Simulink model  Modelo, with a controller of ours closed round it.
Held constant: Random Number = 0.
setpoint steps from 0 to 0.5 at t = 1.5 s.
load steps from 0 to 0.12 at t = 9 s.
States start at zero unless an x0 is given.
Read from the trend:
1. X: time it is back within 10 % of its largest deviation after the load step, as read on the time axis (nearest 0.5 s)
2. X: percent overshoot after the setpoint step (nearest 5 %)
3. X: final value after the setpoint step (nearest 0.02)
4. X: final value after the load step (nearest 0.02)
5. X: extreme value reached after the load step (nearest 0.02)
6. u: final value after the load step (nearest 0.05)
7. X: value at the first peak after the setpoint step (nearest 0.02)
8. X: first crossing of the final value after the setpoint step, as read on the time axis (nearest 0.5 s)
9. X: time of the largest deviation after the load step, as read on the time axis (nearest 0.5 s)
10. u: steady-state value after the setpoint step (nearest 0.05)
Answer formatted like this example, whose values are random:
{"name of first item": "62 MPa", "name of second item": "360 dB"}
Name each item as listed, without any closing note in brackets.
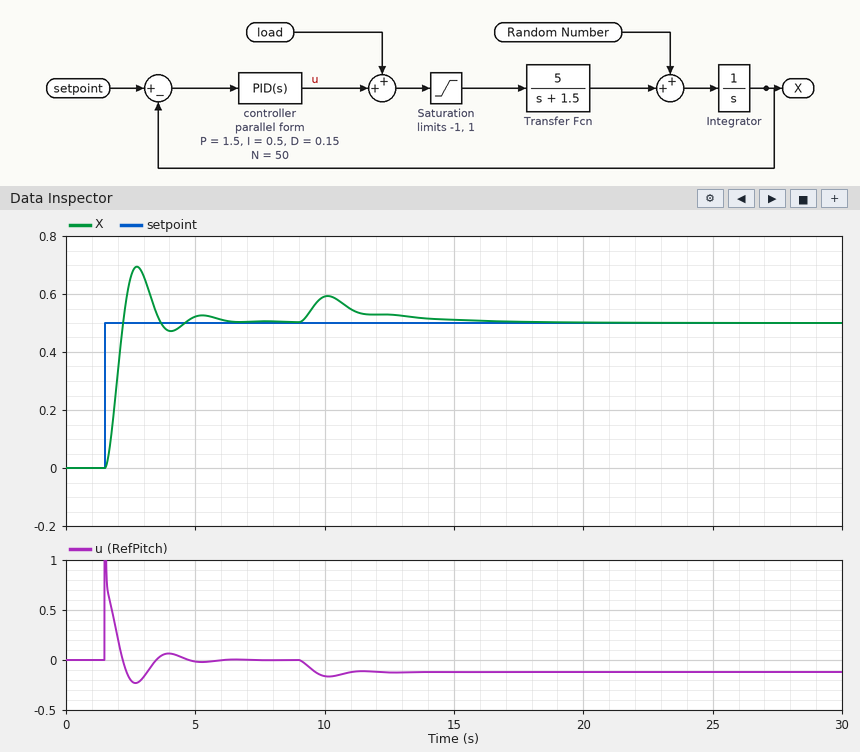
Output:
{"X: time it is back within 10 % of its largest deviation after the load step, as read on the time axis": "15.5 s", "X: percent overshoot after the setpoint step": "40 %", "X: final value after the setpoint step": "0.50", "X: final value after the load step": "0.50", "X: extreme value reached after the load step": "0.60", "u: final value after the load step": "-0.10", "X: value at the first peak after the setpoint step": "0.70", "X: first crossing of the final value after the setpoint step, as read on the time axis": "2.0 s", "X: time of the largest deviation after the load step, as read on the time axis": "10.0 s", "u: steady-state value after the setpoint step": "0.00"}
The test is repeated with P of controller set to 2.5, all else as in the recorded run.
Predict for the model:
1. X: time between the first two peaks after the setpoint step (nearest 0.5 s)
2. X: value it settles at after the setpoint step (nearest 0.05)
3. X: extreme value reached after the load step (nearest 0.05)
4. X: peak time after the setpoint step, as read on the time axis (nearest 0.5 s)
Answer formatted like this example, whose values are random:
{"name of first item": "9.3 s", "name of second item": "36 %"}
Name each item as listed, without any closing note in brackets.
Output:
{"X: time between the first two peaks after the setpoint step": "2.0 s", "X: value it settles at after the setpoint step": "0.50", "X: extreme value reached after the load step": "0.55", "X: peak time after the setpoint step, as read on the time axis": "2.5 s"}
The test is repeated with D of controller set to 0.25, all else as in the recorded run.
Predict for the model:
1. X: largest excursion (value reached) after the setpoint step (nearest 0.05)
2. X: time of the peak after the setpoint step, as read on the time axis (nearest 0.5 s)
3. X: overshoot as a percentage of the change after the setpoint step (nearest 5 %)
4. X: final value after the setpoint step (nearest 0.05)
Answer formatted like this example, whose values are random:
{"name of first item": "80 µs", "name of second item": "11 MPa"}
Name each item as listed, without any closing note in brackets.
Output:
{"X: largest excursion (value reached) after the setpoint step": "0.65", "X: time of the peak after the setpoint step, as read on the time axis": "3.0 s", "X: overshoot as a percentage of the change after the setpoint step": "30 %", "X: final value after the setpoint step": "0.50"}
